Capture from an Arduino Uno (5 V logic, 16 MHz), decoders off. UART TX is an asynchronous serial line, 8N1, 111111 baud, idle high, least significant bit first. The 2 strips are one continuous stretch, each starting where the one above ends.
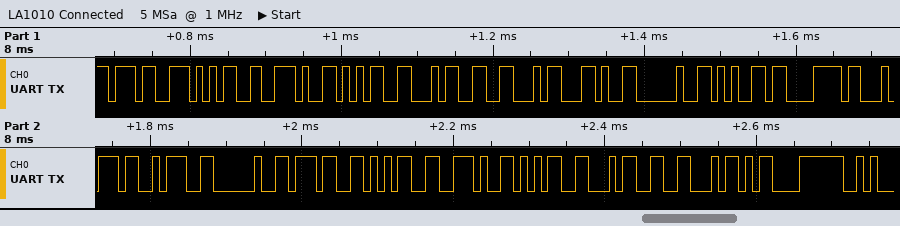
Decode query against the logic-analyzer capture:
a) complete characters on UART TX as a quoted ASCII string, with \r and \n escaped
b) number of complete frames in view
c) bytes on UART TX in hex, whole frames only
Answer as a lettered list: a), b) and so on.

a) "75.54F, ext: 75.54F\r"
b) 20
c) 37 35 2E 35 34 46 2C 20 65 78 74 3A 20 37 35 2E 35 34 46 0D
